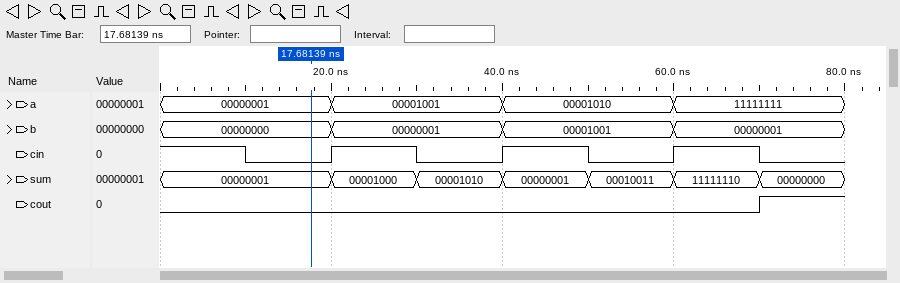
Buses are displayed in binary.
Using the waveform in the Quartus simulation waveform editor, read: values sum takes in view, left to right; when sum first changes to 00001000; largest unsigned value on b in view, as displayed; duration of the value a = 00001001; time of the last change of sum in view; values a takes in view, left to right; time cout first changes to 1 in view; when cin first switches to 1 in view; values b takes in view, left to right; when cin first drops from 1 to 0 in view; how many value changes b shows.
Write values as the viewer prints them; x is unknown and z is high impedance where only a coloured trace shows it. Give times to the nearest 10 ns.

00000001, 00001000, 00001010, 00000001, 00010011, 11111110, 00000000
20 ns
00001001
20 ns
70 ns
00000001, 00001001, 00001010, 11111111
70 ns
20 ns
00000000, 00000001, 00001001, 00000001
10 ns
3
